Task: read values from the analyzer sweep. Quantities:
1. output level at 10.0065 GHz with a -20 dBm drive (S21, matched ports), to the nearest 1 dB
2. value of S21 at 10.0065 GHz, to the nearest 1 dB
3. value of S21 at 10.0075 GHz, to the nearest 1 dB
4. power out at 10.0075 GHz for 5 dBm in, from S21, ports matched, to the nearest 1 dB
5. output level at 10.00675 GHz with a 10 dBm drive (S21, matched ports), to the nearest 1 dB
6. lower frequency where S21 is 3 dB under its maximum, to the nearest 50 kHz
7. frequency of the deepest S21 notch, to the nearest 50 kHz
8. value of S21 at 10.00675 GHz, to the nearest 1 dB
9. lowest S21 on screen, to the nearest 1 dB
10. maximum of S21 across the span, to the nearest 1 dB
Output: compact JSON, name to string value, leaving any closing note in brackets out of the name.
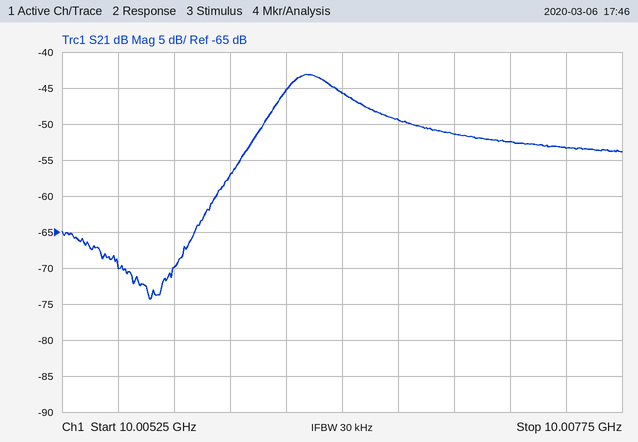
{"output level at 10.0065 GHz with a -20 dBm drive (S21, matched ports), to the nearest 1 dB": "-66 dBm", "value of S21 at 10.0065 GHz, to the nearest 1 dB": "-46 dB", "value of S21 at 10.0075 GHz, to the nearest 1 dB": "-53 dB", "power out at 10.0075 GHz for 5 dBm in, from S21, ports matched, to the nearest 1 dB": "-48 dBm", "output level at 10.00675 GHz with a 10 dBm drive (S21, matched ports), to the nearest 1 dB": "-39 dBm", "lower frequency where S21 is 3 dB under its maximum, to the nearest 50 kHz": "10.00625 GHz", "frequency of the deepest S21 notch, to the nearest 50 kHz": "10.00565 GHz", "value of S21 at 10.00675 GHz, to the nearest 1 dB": "-49 dB", "lowest S21 on screen, to the nearest 1 dB": "-74 dB", "maximum of S21 across the span, to the nearest 1 dB": "-43 dB"}
